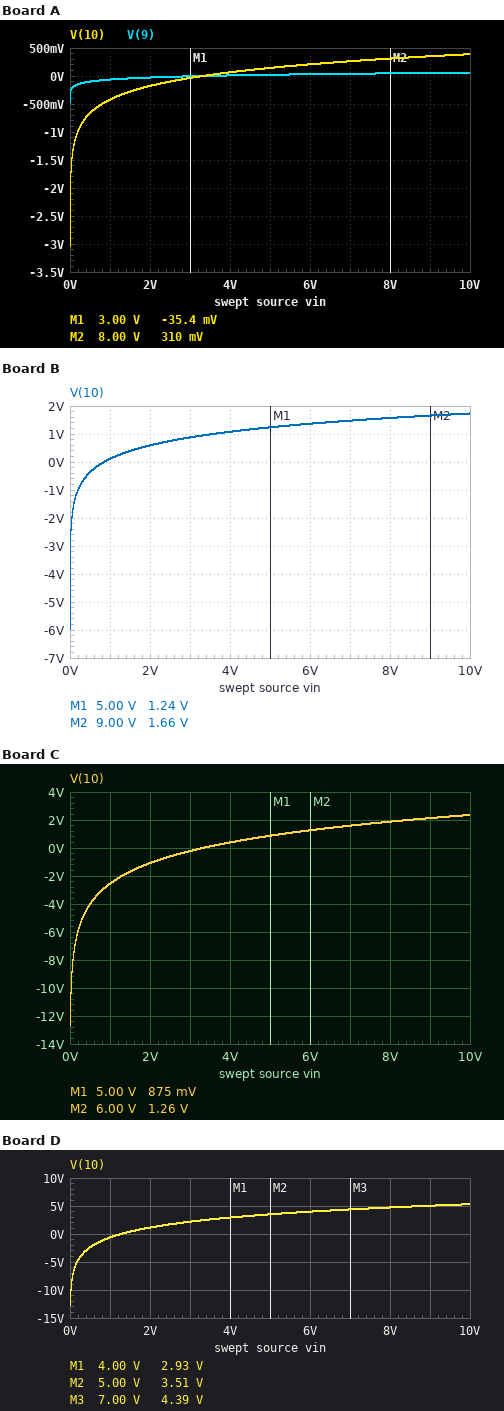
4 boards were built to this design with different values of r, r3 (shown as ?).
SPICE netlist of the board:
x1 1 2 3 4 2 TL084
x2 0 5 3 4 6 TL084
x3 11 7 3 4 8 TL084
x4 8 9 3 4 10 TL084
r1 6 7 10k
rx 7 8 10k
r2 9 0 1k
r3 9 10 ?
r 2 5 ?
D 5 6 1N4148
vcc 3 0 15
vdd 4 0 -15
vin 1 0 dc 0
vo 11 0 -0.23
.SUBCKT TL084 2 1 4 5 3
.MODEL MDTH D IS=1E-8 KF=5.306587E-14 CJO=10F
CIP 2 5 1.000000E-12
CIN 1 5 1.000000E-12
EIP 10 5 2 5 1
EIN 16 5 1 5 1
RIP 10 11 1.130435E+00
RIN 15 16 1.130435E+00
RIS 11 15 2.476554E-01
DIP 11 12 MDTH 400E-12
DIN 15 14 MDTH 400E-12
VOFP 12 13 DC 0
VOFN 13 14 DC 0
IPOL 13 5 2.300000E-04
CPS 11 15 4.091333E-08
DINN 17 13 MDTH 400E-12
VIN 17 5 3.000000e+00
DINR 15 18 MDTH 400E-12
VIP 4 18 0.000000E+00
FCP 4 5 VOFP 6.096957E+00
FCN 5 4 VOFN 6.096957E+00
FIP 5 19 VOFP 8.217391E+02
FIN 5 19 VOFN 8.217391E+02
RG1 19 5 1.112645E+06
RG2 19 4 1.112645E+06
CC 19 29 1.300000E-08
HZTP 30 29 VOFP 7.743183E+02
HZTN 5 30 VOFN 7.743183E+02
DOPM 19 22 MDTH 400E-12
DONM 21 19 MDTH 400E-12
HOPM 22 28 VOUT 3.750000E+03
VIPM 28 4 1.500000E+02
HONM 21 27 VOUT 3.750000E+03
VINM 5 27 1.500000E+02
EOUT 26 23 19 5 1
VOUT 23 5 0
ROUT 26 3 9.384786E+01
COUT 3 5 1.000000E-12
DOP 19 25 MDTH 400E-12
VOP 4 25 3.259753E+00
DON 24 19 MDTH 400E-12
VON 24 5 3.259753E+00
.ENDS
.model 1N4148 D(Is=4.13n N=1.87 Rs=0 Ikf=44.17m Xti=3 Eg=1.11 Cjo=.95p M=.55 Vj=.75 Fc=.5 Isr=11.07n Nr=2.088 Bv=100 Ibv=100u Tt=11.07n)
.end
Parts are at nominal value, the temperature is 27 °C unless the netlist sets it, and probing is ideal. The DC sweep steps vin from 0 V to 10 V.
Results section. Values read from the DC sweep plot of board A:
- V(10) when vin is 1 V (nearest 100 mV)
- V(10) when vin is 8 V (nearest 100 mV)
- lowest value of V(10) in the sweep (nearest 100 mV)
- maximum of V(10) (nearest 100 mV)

-400 mV
300 mV
-3.0 V
400 mV
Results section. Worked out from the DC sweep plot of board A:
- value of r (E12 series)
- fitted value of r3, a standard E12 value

39 kΩ
5.6 kΩ
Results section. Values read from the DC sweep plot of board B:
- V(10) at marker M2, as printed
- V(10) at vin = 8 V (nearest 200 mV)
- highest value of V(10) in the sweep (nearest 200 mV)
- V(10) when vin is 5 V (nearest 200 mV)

1.66 V
1.6 V
1.8 V
1.2 V
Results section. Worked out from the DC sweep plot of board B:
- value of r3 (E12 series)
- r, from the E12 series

12 kΩ
10 kΩ
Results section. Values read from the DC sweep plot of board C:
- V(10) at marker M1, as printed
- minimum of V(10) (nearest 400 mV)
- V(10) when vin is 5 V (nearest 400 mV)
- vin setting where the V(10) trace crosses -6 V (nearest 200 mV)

875 mV
-12.8 V
800 mV
200 mV
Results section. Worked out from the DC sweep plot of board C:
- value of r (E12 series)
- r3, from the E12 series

39 kΩ
39 kΩ
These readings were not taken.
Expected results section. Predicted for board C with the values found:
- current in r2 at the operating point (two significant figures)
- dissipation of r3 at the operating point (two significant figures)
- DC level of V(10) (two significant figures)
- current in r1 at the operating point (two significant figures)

320 µA
3.9 mW
-13 V
23 µA
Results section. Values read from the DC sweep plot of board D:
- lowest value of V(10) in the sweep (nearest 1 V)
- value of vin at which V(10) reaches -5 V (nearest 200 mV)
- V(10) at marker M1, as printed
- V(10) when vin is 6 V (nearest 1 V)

-13 V
200 mV
2.93 V
4 V
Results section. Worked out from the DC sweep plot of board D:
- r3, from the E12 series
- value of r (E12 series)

47 kΩ
15 kΩ
